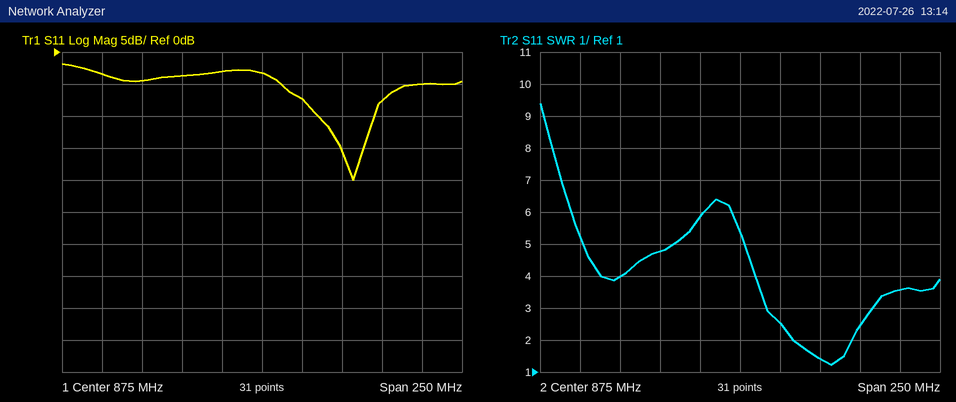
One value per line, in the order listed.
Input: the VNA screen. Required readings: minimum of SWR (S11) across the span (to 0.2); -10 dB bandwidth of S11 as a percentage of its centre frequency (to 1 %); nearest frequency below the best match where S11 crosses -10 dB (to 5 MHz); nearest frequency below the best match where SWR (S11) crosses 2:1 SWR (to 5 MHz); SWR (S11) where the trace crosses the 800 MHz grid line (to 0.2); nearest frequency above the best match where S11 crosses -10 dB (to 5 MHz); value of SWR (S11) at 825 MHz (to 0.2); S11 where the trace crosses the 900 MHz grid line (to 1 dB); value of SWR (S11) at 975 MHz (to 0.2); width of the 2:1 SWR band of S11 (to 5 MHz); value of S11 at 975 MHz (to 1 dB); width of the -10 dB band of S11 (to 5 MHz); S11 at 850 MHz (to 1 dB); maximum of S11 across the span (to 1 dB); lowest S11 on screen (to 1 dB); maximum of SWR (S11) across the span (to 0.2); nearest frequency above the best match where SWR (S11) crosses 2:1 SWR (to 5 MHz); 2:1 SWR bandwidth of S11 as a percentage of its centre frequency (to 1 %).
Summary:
1.2
4 %
910 MHz
910 MHz
4.0
945 MHz
4.8
-7 dB
3.6
35 MHz
-5 dB
35 MHz
-3 dB
-2 dB
-20 dB
9.4
945 MHz
4 %
